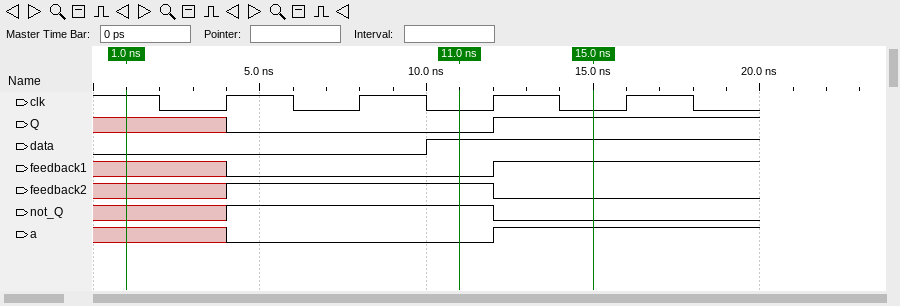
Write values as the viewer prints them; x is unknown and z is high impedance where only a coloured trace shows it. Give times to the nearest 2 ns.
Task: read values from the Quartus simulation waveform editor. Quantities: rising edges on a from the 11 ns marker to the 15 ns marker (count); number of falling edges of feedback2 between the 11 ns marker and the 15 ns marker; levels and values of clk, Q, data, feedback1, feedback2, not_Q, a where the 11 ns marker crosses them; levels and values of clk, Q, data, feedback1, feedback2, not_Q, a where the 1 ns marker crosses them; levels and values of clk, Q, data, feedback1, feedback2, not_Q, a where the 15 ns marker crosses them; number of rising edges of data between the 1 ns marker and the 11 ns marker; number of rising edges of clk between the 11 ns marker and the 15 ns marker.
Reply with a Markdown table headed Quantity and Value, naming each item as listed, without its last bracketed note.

| Quantity | Value |
|---|---|
| rising edges on a from the 11 ns marker to the 15 ns marker | 1 |
| number of falling edges of feedback2 between the 11 ns marker and the 15 ns marker | 1 |
| levels and values of clk, Q, data, feedback1, feedback2, not_Q, a where the 11 ns marker crosses them | clk=0, Q=0, data=1, feedback1=0, feedback2=1, not_Q=1, a=0 |
| levels and values of clk, Q, data, feedback1, feedback2, not_Q, a where the 1 ns marker crosses them | clk=1, Q=x, data=0, feedback1=x, feedback2=x, not_Q=x, a=x |
| levels and values of clk, Q, data, feedback1, feedback2, not_Q, a where the 15 ns marker crosses them | clk=0, Q=1, data=1, feedback1=1, feedback2=0, not_Q=0, a=1 |
| number of rising edges of data between the 1 ns marker and the 11 ns marker | 1 |
| number of rising edges of clk between the 11 ns marker and the 15 ns marker | 1 |
